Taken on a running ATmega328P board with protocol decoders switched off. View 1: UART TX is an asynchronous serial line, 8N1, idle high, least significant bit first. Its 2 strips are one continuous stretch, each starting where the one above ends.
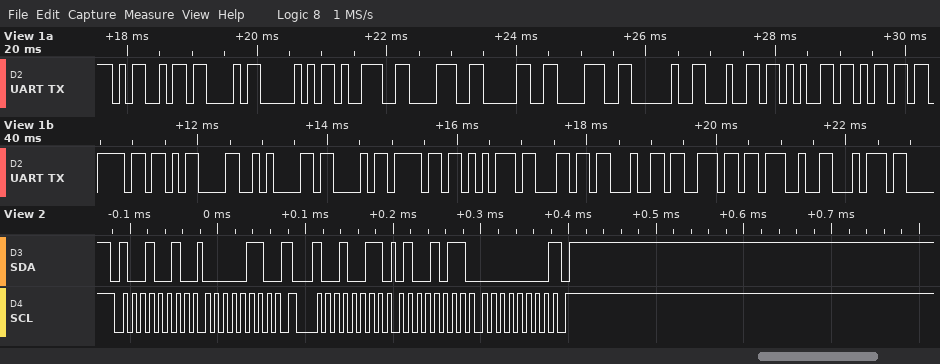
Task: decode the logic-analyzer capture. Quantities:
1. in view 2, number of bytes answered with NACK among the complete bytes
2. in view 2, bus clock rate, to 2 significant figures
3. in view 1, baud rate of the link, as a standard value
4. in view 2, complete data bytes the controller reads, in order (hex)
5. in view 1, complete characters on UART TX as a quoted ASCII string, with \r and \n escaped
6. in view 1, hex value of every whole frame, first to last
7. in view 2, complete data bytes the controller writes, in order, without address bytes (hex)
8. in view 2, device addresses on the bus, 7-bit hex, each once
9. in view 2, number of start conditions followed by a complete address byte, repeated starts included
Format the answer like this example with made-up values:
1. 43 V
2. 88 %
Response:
1. 1
2. 100 kHz
3. 9600 baud
4. 4B 00
5. "MCP9808 demo\r\nCouldn't"
6. 4D 43 50 39 38 30 38 20 64 65 6D 6F 0D 0A 43 6F 75 6C 64 6E 27 74
7. 06
8. 0x49
9. 2
